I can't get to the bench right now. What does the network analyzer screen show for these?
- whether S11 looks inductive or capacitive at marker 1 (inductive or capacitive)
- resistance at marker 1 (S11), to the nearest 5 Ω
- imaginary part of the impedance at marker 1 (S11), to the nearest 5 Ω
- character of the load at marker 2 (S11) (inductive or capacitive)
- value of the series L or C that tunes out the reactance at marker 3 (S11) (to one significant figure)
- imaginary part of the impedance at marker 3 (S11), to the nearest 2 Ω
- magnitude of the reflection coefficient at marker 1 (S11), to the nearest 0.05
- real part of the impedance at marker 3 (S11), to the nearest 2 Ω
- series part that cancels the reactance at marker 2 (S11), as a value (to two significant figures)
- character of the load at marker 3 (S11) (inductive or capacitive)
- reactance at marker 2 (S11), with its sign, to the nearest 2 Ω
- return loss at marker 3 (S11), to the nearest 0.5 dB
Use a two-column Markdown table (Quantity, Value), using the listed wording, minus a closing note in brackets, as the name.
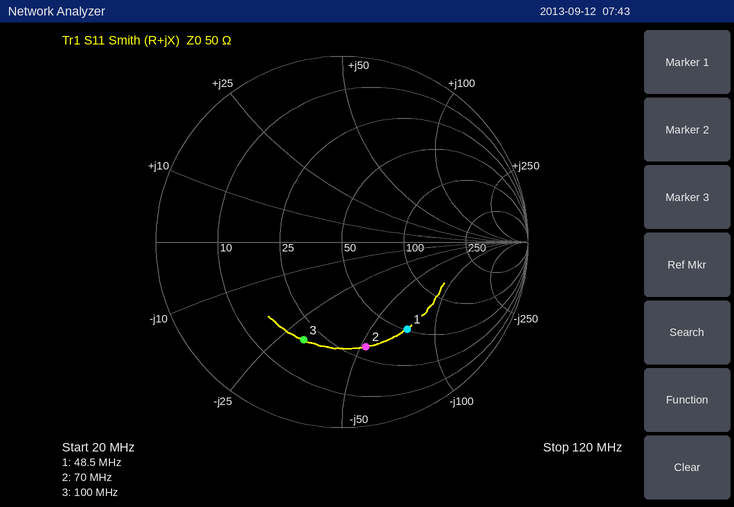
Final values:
| Quantity | Value |
|---|---|
| whether S11 looks inductive or capacitive at marker 1 | capacitive |
| resistance at marker 1 (S11), to the nearest 5 Ω | 50 Ω |
| imaginary part of the impedance at marker 1 (S11), to the nearest 5 Ω | -75 Ω |
| character of the load at marker 2 (S11) | capacitive |
| value of the series L or C that tunes out the reactance at marker 3 (S11) | 50 nH |
| imaginary part of the impedance at marker 3 (S11), to the nearest 2 Ω | -30 Ω |
| magnitude of the reflection coefficient at marker 1 (S11), to the nearest 0.05 | 0.60 |
| real part of the impedance at marker 3 (S11), to the nearest 2 Ω | 20 Ω |
| series part that cancels the reactance at marker 2 (S11), as a value | 120 nH |
| character of the load at marker 3 (S11) | capacitive |
| reactance at marker 2 (S11), with its sign, to the nearest 2 Ω | -52 Ω |
| return loss at marker 3 (S11), to the nearest 0.5 dB | 5.0 dB |
